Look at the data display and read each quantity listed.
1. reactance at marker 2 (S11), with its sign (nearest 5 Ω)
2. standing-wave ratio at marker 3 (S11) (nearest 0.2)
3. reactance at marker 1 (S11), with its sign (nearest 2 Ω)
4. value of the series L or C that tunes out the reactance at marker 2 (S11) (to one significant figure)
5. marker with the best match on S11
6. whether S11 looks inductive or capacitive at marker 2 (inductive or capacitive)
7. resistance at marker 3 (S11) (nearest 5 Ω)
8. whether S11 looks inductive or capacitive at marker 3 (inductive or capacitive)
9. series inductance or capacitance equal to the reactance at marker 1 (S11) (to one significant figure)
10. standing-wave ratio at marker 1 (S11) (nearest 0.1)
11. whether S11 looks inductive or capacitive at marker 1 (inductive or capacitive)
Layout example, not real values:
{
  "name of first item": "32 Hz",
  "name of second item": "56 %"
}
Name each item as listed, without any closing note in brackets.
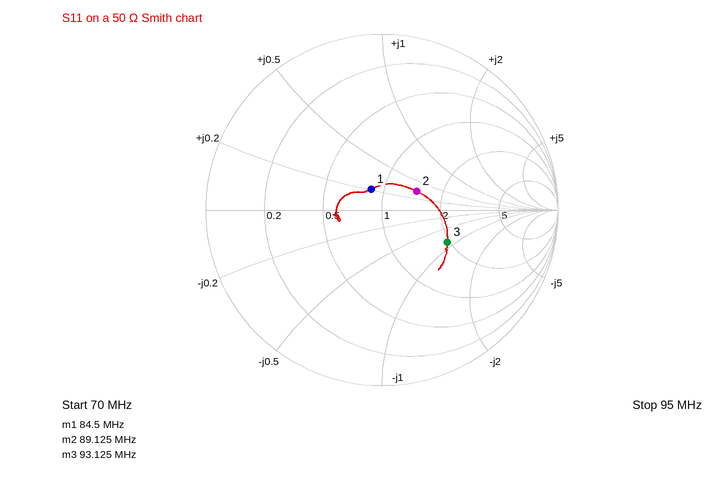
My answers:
{
  "reactance at marker 2 (S11), with its sign": "+15 Ω",
  "standing-wave ratio at marker 3 (S11)": "2.4",
  "reactance at marker 1 (S11), with its sign": "+10 Ω",
  "value of the series L or C that tunes out the reactance at marker 2 (S11)": "100 pF",
  "marker with the best match on S11": "marker 1",
  "whether S11 looks inductive or capacitive at marker 2": "inductive",
  "resistance at marker 3 (S11)": "95 Ω",
  "whether S11 looks inductive or capacitive at marker 3": "capacitive",
  "series inductance or capacitance equal to the reactance at marker 1 (S11)": "20 nH",
  "standing-wave ratio at marker 1 (S11)": "1.3",
  "whether S11 looks inductive or capacitive at marker 1": "inductive"
}
